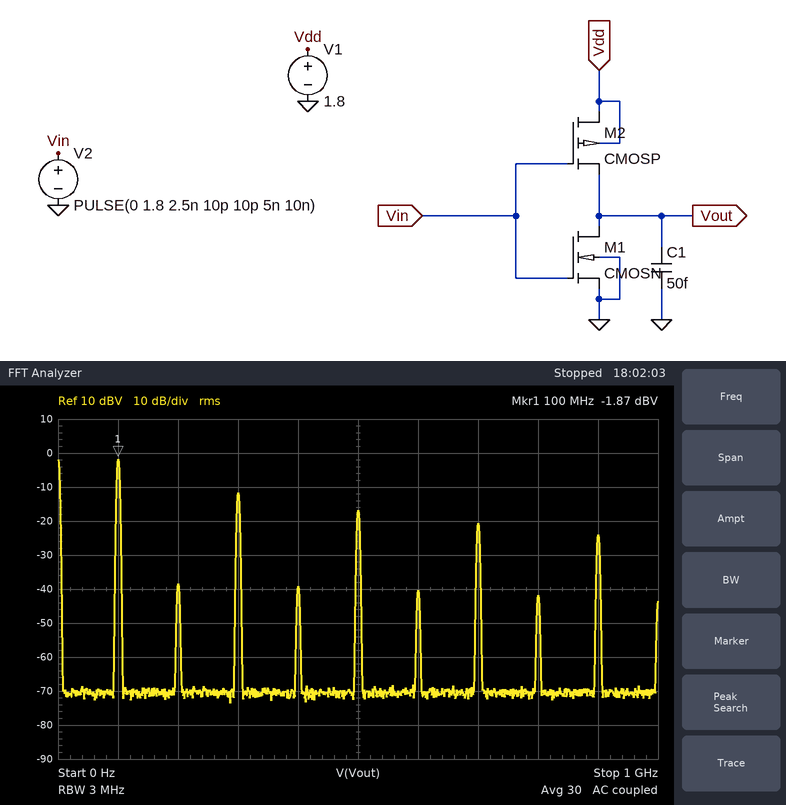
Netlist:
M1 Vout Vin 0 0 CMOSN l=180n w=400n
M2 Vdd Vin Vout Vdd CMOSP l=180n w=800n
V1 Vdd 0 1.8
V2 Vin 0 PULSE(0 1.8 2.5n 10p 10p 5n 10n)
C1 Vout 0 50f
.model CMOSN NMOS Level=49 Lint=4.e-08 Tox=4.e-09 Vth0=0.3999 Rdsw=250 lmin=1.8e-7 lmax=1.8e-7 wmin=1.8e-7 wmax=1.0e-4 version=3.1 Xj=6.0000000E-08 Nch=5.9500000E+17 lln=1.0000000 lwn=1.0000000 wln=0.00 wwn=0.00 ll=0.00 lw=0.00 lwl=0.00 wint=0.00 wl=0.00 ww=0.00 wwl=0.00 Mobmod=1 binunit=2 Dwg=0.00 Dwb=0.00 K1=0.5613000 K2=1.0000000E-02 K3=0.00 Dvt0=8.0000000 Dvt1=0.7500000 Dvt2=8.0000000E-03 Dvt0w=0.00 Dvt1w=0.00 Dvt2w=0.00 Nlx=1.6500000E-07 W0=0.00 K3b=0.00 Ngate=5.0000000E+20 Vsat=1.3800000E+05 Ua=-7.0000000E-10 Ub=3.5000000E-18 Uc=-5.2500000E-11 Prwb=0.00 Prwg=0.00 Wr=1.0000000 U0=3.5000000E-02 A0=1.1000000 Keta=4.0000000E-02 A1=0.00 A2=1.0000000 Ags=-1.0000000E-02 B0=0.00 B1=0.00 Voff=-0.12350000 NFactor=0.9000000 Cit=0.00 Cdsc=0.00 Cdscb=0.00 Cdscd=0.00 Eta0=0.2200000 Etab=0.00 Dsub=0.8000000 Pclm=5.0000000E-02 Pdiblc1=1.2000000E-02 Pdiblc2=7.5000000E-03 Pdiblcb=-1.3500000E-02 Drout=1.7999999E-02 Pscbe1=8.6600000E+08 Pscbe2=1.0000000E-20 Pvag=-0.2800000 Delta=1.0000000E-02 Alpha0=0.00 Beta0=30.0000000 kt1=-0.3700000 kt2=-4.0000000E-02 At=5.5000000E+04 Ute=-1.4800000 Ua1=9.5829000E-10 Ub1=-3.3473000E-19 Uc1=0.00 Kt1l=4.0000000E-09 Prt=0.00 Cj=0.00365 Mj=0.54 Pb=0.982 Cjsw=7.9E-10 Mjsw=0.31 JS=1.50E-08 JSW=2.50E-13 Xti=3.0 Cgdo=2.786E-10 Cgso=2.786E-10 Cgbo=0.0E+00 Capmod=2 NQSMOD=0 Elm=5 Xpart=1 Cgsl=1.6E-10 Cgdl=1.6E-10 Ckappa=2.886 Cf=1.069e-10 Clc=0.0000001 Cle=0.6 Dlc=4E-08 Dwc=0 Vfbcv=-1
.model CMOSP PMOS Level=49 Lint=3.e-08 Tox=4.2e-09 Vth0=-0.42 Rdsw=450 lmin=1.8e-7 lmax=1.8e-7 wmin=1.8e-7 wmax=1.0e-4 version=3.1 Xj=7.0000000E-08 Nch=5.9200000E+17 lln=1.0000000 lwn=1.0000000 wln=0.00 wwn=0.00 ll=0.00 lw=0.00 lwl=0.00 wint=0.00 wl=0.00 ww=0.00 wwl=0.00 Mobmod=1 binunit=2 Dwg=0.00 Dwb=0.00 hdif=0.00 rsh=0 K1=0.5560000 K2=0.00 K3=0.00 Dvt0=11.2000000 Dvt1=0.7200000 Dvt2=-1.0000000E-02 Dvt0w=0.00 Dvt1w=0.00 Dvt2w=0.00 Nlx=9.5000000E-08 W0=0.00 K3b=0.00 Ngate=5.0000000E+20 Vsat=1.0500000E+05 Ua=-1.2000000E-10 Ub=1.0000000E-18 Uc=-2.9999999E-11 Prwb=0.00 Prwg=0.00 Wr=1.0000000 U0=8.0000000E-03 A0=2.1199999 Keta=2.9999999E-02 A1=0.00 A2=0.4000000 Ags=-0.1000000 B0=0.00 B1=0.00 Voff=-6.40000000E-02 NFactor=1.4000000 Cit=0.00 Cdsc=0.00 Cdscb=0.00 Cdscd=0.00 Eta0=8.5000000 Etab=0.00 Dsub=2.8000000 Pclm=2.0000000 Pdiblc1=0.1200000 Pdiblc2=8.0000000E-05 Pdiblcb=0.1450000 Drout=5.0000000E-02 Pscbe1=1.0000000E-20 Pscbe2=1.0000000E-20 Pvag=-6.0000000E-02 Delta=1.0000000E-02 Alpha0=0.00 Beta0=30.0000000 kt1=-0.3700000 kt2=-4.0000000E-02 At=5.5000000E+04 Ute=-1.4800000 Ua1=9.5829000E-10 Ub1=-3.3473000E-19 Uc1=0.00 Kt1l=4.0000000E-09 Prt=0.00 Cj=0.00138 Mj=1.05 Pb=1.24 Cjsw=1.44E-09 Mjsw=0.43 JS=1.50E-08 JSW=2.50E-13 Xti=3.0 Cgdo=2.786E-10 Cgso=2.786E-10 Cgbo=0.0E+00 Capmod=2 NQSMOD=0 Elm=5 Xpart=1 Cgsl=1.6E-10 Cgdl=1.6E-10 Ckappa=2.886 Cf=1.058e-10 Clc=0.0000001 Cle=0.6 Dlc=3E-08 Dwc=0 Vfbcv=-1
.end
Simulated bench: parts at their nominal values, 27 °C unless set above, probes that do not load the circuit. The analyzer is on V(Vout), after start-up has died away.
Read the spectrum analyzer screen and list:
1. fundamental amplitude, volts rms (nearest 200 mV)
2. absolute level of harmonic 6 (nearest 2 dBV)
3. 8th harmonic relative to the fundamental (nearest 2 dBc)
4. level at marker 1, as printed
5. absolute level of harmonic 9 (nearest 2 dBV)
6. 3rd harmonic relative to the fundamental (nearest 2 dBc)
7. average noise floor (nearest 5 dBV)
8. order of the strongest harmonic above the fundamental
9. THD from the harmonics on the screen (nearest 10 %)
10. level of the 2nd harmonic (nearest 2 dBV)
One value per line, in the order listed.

800 mV
-40 dBV
-40 dBc
-1.87 dBV
-24 dBV
-10 dBc
-70 dBV
3
40 %
-38 dBV
